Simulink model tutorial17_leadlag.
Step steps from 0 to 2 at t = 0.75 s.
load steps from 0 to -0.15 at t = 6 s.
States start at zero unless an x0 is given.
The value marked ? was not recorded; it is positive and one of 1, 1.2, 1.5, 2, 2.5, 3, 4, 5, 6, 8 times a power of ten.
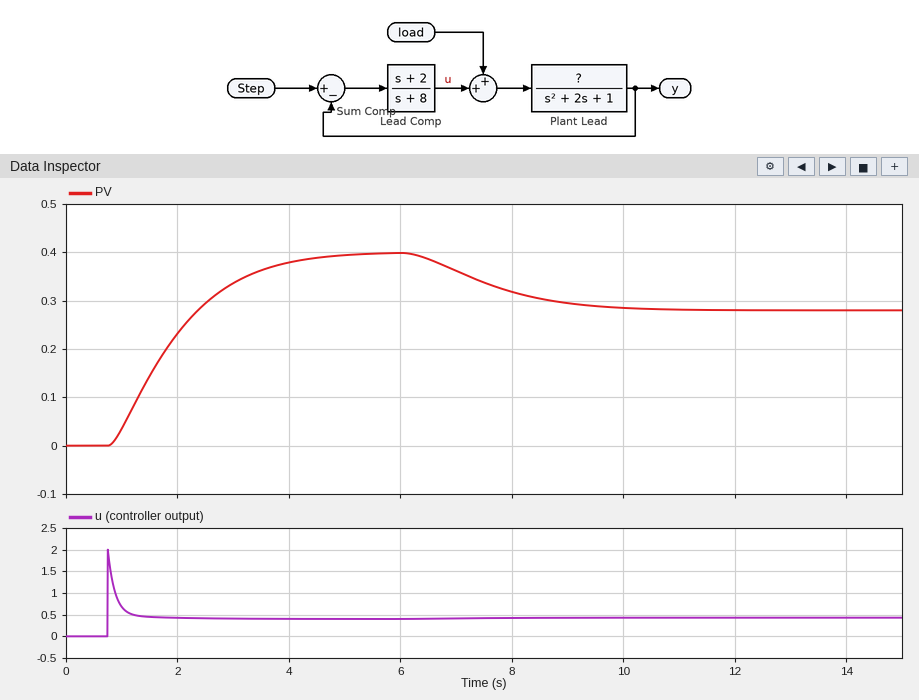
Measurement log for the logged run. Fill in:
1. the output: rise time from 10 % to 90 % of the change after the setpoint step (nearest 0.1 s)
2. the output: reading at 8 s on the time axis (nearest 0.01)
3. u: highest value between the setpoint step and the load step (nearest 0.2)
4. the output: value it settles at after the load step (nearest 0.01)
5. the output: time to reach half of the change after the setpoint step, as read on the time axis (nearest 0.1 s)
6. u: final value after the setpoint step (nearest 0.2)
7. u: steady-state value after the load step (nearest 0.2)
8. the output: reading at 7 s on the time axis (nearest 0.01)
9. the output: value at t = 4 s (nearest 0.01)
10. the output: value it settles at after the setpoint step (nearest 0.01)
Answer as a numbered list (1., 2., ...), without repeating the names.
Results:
1. 2.4 s
2. 0.32
3. 2.0
4. 0.28
5. 1.8 s
6. 0.4
7. 0.4
8. 0.36
9. 0.38
10. 0.40
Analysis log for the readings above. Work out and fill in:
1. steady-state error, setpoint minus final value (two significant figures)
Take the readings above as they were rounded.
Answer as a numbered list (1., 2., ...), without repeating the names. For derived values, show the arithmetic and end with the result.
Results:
1. 2 - 0.4 = 1.6
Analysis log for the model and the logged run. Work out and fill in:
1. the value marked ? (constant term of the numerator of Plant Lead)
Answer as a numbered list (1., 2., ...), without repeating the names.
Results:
1. 1
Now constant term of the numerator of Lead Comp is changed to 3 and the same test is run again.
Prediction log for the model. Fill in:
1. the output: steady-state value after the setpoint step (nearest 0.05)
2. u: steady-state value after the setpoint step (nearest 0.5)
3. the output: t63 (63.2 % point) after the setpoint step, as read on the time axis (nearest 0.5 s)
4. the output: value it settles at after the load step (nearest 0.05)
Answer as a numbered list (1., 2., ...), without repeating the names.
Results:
1. 0.55
2. 0.5
3. 2.0 s
4. 0.45
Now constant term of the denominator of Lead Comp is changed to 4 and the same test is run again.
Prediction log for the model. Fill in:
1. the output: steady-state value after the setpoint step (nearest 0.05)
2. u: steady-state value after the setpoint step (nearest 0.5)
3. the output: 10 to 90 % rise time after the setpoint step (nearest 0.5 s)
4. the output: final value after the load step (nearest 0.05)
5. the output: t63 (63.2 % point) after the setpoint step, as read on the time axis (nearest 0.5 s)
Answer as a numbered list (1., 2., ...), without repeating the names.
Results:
1. 0.65
2. 0.5
3. 2.0 s
4. 0.55
5. 2.0 s
